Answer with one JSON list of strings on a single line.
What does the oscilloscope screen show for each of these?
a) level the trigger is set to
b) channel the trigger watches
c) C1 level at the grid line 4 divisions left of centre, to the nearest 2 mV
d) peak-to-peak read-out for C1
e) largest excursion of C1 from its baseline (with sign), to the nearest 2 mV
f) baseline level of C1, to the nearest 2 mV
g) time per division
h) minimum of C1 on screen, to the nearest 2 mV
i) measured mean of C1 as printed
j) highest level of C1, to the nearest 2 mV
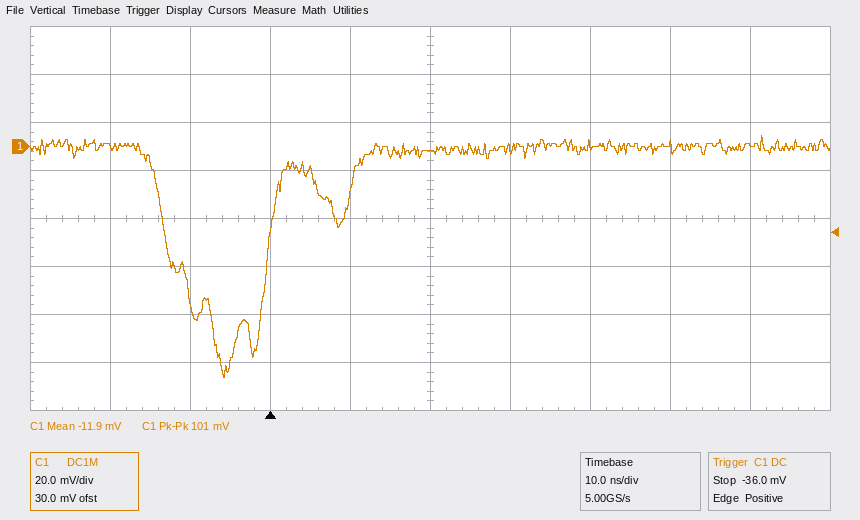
["-36.0 mV", "C1", "0 mV", "101 mV", "-96 mV", "0 mV", "10 ns", "-96 mV", "-11.9 mV", "4 mV"]
